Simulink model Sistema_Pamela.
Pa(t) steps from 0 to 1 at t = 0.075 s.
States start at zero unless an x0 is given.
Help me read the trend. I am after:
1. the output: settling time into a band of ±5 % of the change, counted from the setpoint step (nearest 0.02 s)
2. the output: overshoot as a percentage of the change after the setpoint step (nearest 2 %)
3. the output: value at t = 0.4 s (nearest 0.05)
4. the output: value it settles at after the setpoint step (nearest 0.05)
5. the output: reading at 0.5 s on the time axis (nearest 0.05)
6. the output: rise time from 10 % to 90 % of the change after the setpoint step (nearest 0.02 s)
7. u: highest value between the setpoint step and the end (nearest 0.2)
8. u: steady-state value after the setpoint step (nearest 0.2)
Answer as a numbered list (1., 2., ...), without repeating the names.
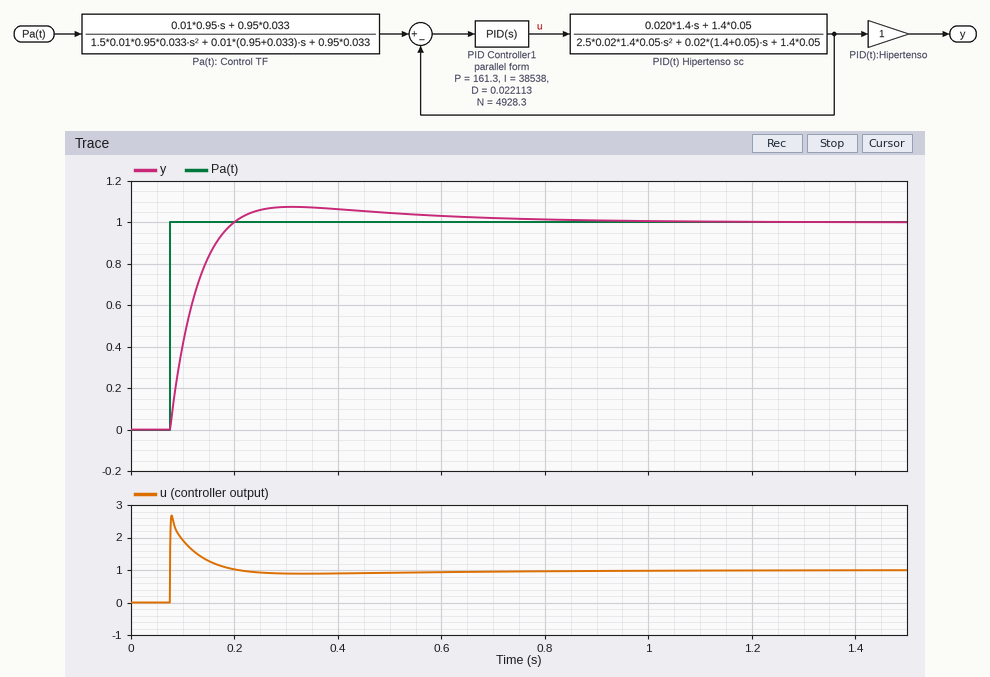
1. 0.40 s
2. 8 %
3. 1.05
4. 1.00
5. 1.05
6. 0.08 s
7. 2.6
8. 1.0
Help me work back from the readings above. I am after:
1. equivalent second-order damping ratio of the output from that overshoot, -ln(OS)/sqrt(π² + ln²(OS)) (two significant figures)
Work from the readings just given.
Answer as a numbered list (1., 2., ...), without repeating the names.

1. 0.63
